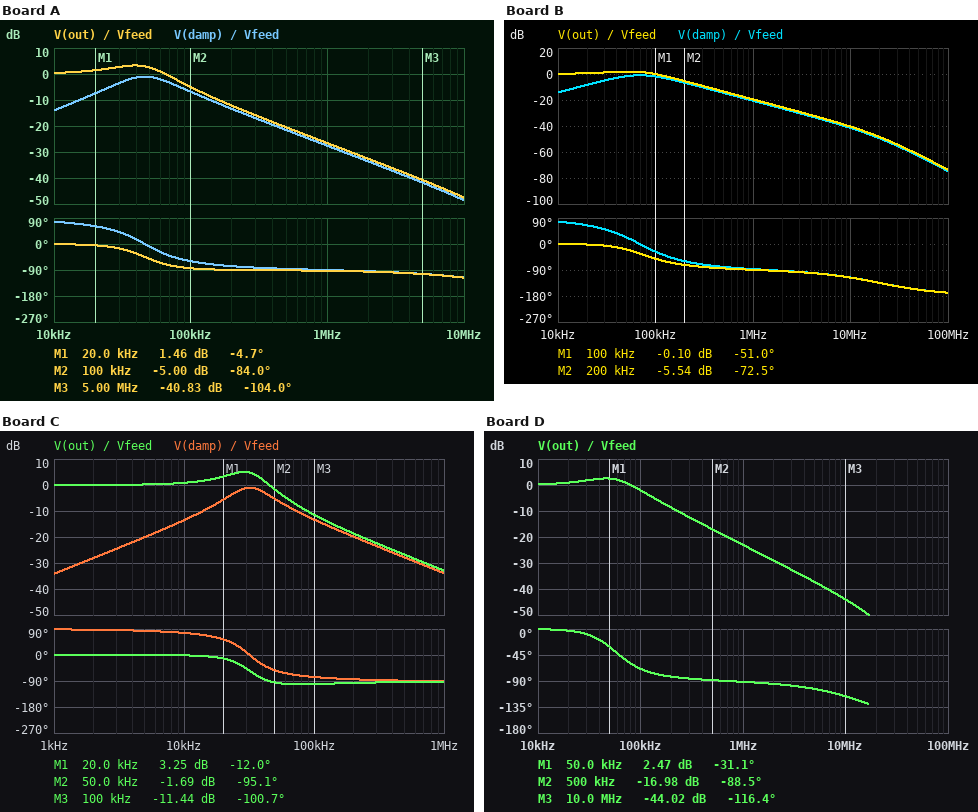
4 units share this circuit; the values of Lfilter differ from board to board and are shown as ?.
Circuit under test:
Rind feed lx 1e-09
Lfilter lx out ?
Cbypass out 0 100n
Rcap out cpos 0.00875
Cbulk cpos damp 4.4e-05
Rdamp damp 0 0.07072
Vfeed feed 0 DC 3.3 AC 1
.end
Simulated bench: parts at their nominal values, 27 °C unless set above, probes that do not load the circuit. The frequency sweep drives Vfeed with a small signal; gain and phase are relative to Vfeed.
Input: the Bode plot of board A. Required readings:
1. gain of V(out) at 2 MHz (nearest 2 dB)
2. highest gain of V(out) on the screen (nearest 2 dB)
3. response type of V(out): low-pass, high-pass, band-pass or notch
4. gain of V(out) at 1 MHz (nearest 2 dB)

-32 dB
4 dB
low-pass
-26 dB
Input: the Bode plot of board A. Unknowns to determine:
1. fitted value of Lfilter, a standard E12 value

270 nH
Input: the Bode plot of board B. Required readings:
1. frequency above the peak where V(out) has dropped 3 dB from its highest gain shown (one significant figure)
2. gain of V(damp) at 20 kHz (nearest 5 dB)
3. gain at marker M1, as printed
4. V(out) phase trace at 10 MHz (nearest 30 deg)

100 kHz
-10 dB
-0.10 dB
-120 deg
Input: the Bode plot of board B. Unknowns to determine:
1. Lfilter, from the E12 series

120 nH
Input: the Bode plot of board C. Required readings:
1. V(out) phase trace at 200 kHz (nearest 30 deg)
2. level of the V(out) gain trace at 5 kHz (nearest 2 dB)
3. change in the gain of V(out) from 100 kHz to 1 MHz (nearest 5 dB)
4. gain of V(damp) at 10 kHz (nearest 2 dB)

-90 deg
0 dB
-20 dB
-14 dB
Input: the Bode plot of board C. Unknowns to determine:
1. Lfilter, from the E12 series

560 nH
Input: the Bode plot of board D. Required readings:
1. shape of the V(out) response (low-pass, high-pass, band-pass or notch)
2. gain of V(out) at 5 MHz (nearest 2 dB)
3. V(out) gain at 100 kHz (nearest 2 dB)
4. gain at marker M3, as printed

low-pass
-38 dB
-2 dB
-44.02 dB
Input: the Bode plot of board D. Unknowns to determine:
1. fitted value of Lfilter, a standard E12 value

180 nH
